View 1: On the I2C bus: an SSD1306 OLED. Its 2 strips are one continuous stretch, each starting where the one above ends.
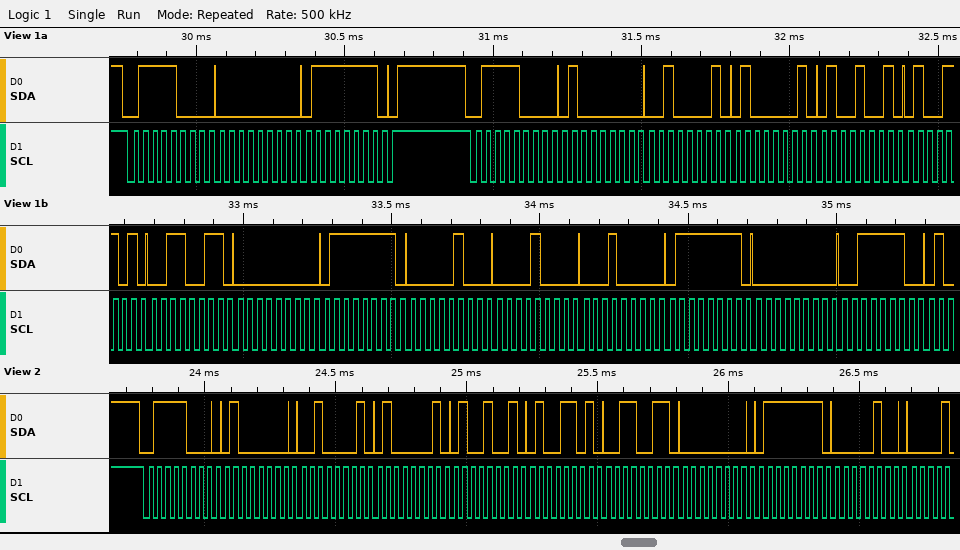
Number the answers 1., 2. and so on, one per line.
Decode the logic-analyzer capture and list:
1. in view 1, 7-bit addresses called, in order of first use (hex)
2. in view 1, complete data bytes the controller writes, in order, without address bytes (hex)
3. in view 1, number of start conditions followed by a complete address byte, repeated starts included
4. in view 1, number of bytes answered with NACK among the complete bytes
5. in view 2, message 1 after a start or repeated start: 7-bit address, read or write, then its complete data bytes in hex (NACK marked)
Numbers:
1. 0x3C
2. 00 7F 40 21 41 49 4D 33 00 7F 04 08 10 7F 00 3E
3. 2
4. 0
5. 0x3C write: 40 21 41 49 4D 33 00 7F 04
